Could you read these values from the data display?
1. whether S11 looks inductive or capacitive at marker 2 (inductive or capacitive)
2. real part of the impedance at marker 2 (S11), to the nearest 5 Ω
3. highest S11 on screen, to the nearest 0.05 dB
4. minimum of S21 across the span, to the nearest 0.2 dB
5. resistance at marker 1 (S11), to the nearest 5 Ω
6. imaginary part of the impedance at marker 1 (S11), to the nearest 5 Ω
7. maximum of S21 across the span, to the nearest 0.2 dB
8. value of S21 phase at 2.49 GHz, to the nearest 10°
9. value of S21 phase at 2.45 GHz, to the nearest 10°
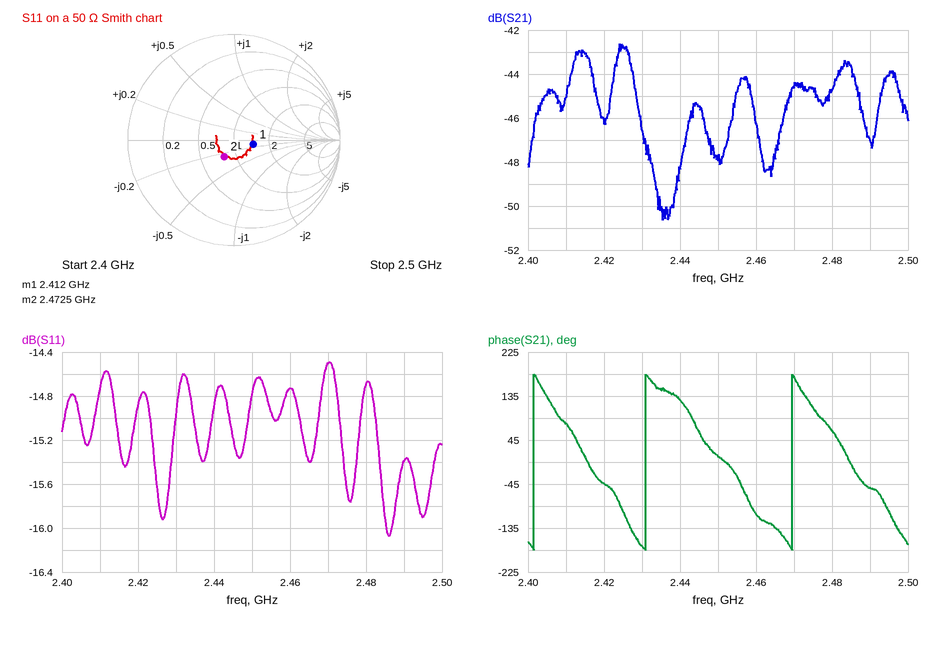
capacitive
40 Ω
-14.50 dB
-50.6 dB
70 Ω
-5 Ω
-42.6 dB
-50°
10°
